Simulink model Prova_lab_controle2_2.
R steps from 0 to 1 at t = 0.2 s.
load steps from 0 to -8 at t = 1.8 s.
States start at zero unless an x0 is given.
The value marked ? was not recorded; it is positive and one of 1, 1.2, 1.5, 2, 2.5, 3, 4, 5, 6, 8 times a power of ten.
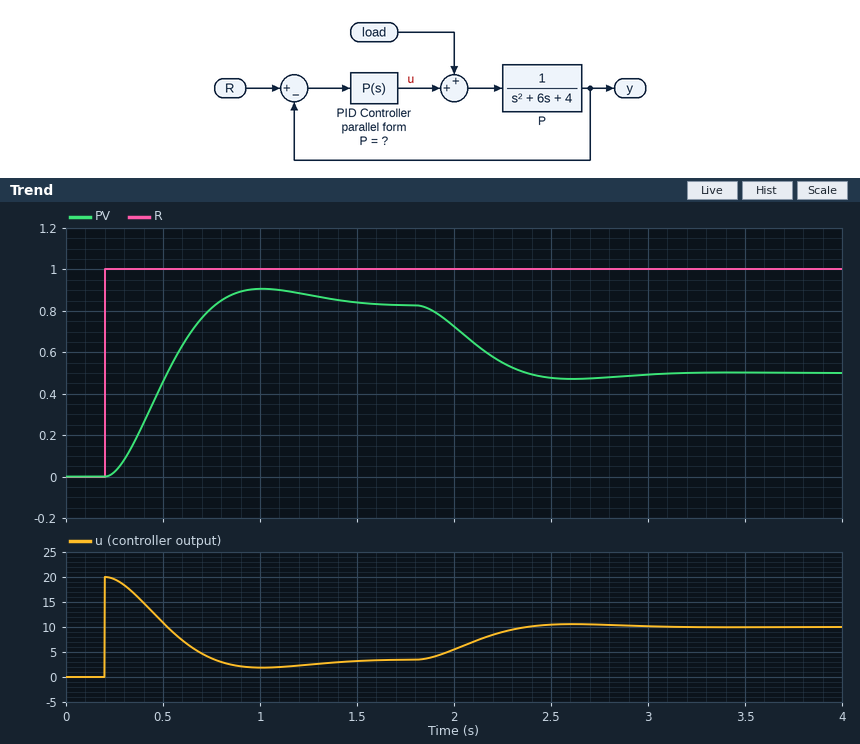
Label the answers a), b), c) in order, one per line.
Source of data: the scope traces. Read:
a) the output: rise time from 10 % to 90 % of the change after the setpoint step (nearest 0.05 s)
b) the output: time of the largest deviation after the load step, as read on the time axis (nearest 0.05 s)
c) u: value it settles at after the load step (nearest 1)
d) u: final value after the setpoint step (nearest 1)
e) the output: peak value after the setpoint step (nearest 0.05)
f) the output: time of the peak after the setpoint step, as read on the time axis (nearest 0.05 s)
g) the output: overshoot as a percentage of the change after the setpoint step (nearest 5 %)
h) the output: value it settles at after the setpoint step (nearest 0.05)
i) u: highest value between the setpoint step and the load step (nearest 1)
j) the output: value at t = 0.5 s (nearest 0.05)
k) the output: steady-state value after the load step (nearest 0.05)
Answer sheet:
a) 0.40 s
b) 2.60 s
c) 10
d) 3
e) 0.90
f) 1.00 s
g) 10 %
h) 0.85
i) 20
j) 0.45
k) 0.50
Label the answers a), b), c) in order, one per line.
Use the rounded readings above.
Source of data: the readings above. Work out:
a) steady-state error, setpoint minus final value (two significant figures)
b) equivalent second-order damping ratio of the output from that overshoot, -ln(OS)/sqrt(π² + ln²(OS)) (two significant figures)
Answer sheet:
a) 0.15
b) 0.59
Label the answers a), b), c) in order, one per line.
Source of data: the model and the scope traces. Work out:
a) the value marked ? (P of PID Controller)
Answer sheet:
a) 20
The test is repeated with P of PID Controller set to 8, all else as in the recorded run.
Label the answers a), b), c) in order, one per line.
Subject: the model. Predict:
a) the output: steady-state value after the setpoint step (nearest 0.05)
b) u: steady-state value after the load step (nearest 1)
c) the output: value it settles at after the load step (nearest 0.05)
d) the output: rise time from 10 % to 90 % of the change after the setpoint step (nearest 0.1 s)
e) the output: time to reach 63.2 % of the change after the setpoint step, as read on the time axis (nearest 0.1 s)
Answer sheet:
a) 0.65
b) 8
c) 0.00
d) 0.8 s
e) 0.8 s
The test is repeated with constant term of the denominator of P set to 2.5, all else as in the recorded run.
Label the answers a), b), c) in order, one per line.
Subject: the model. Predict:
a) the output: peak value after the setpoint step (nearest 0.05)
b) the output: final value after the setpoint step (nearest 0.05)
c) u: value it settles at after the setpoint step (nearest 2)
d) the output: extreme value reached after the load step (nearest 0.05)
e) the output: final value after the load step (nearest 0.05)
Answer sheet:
a) 0.95
b) 0.90
c) 2
d) 0.50
e) 0.55
